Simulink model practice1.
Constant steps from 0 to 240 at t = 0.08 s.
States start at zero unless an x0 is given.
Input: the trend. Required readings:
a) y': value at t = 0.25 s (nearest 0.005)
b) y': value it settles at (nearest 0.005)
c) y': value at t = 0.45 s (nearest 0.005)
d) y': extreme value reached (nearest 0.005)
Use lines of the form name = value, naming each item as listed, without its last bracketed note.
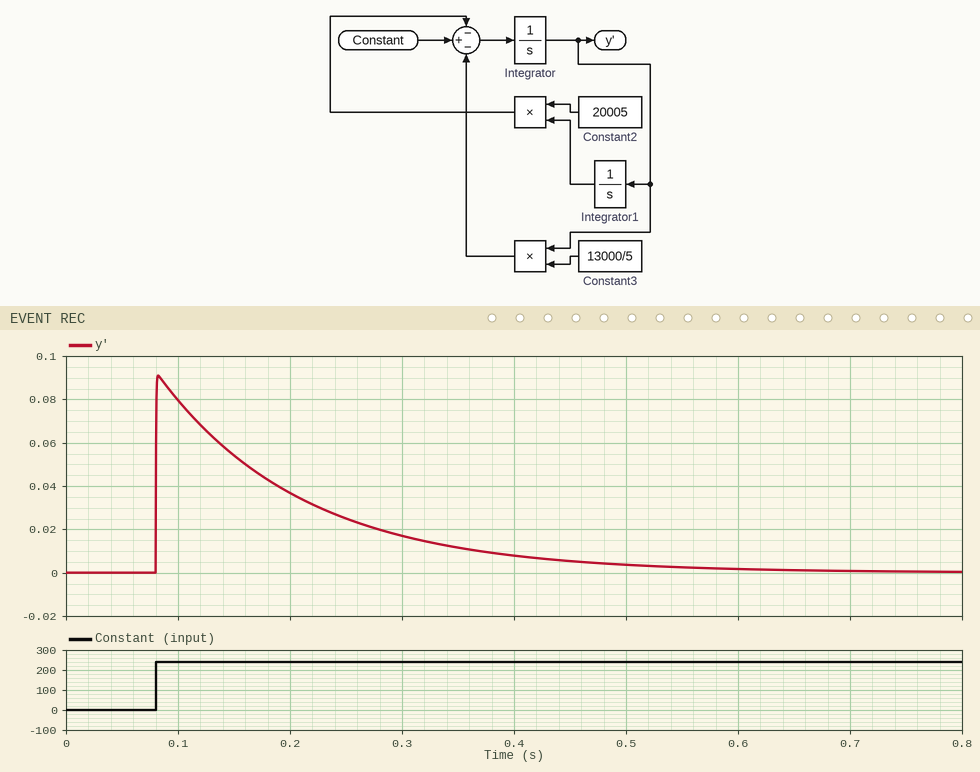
y': value at t = 0.25 s = 0.025
y': value it settles at = 0.000
y': value at t = 0.45 s = 0.005
y': extreme value reached = 0.090
